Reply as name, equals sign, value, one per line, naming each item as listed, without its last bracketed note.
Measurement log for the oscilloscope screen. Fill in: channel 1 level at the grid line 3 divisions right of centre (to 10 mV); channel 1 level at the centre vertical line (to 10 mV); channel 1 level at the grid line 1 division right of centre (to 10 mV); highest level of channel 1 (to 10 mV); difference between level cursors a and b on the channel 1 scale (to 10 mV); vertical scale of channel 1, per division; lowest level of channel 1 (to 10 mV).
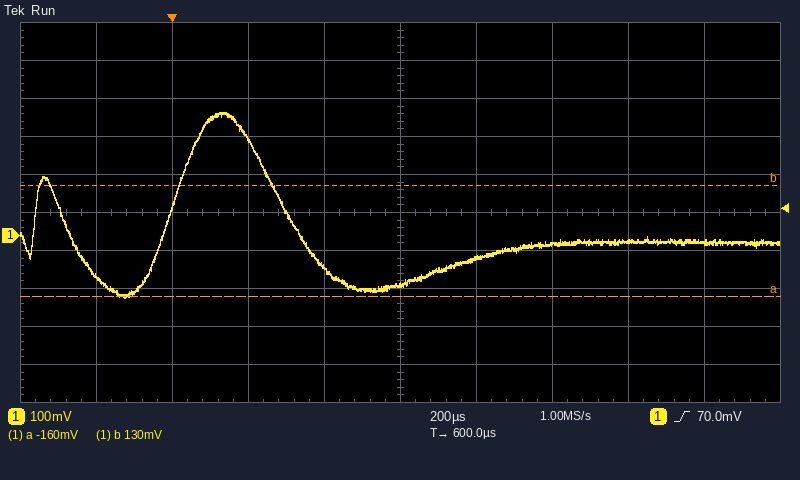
channel 1 level at the grid line 3 divisions right of centre = -20 mV
channel 1 level at the centre vertical line = -130 mV
channel 1 level at the grid line 1 division right of centre = -60 mV
highest level of channel 1 = 320 mV
difference between level cursors a and b on the channel 1 scale = 290 mV
vertical scale of channel 1, per division = 100 mV
lowest level of channel 1 = -160 mV
